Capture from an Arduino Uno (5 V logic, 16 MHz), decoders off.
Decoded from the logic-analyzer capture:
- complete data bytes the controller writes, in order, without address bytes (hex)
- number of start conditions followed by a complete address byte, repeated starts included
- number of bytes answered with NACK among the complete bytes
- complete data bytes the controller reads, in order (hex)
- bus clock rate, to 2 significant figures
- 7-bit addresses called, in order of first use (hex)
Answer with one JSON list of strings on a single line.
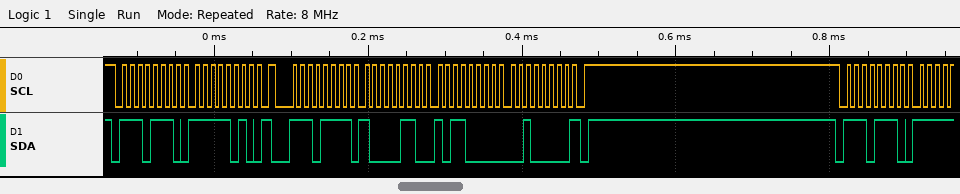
["FA", "3", "1", "86 B0 20", "100 kHz", "0x77"]
